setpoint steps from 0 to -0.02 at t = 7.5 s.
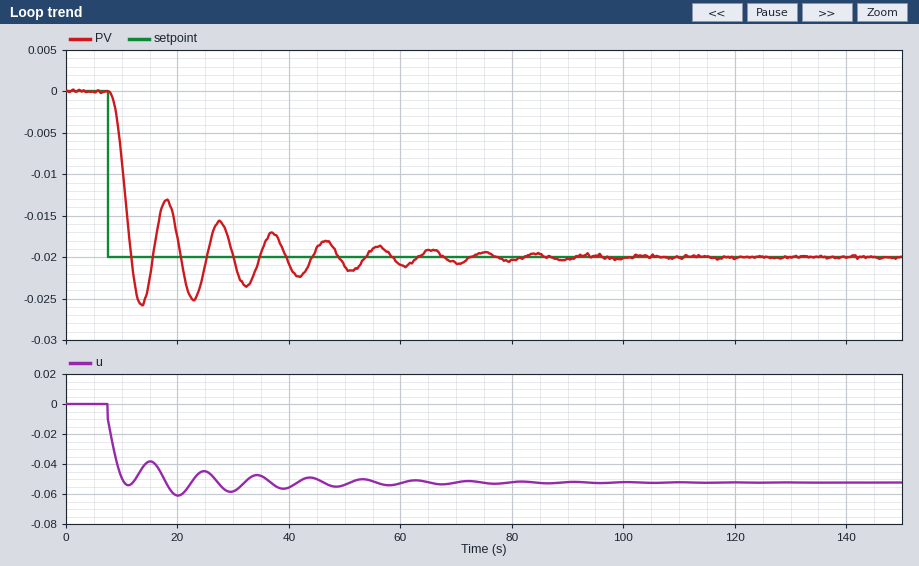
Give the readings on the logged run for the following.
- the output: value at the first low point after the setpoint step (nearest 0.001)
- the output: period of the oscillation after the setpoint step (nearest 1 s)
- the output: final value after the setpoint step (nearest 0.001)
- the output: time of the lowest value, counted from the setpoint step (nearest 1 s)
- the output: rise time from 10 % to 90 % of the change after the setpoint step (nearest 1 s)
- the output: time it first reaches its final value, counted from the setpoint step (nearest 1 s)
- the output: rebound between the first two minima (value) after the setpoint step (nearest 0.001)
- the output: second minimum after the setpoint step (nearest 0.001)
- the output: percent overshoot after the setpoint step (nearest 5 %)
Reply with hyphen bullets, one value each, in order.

- -0.026
- 9 s
- -0.020
- 6 s
- 3 s
- 4 s
- -0.013
- -0.025
- 30 %
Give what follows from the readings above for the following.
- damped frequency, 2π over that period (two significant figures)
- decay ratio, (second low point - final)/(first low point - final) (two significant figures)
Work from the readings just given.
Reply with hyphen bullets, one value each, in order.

- 0.70 rad/s
- 0.83
